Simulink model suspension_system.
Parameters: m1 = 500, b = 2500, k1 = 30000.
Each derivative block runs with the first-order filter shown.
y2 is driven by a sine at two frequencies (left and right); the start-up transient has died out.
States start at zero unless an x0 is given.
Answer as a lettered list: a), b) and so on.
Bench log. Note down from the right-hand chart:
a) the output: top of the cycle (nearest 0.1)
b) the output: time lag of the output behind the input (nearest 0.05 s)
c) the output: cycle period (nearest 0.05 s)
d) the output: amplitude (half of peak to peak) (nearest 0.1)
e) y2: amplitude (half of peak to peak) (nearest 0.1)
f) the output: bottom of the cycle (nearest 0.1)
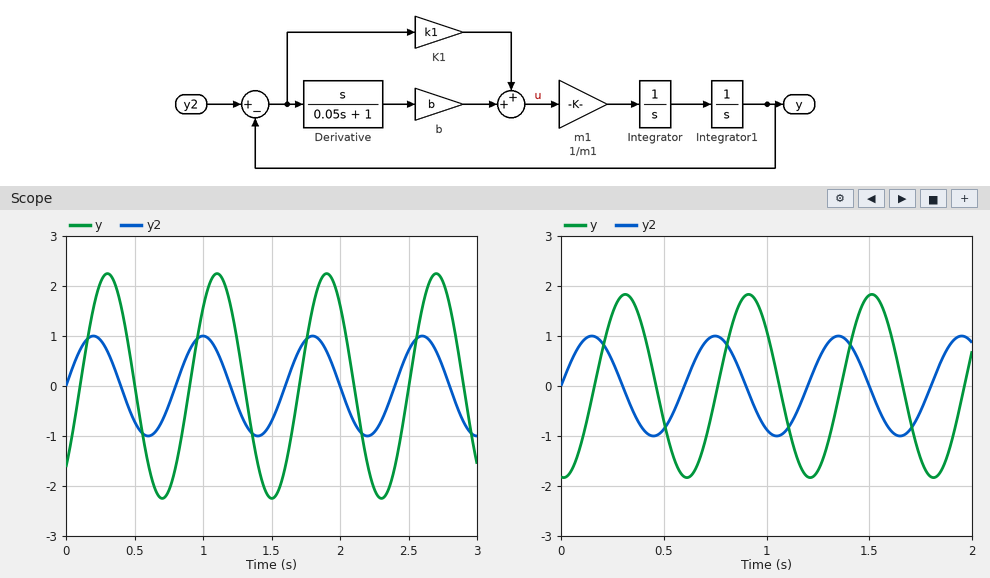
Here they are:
a) 1.8
b) 0.15 s
c) 0.60 s
d) 1.8
e) 1.0
f) -1.8
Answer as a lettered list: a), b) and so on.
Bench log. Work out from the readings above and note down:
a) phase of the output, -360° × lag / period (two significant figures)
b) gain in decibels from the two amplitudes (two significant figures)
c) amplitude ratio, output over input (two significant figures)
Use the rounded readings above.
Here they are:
a) -90°
b) 5.1 dB
c) 1.8
